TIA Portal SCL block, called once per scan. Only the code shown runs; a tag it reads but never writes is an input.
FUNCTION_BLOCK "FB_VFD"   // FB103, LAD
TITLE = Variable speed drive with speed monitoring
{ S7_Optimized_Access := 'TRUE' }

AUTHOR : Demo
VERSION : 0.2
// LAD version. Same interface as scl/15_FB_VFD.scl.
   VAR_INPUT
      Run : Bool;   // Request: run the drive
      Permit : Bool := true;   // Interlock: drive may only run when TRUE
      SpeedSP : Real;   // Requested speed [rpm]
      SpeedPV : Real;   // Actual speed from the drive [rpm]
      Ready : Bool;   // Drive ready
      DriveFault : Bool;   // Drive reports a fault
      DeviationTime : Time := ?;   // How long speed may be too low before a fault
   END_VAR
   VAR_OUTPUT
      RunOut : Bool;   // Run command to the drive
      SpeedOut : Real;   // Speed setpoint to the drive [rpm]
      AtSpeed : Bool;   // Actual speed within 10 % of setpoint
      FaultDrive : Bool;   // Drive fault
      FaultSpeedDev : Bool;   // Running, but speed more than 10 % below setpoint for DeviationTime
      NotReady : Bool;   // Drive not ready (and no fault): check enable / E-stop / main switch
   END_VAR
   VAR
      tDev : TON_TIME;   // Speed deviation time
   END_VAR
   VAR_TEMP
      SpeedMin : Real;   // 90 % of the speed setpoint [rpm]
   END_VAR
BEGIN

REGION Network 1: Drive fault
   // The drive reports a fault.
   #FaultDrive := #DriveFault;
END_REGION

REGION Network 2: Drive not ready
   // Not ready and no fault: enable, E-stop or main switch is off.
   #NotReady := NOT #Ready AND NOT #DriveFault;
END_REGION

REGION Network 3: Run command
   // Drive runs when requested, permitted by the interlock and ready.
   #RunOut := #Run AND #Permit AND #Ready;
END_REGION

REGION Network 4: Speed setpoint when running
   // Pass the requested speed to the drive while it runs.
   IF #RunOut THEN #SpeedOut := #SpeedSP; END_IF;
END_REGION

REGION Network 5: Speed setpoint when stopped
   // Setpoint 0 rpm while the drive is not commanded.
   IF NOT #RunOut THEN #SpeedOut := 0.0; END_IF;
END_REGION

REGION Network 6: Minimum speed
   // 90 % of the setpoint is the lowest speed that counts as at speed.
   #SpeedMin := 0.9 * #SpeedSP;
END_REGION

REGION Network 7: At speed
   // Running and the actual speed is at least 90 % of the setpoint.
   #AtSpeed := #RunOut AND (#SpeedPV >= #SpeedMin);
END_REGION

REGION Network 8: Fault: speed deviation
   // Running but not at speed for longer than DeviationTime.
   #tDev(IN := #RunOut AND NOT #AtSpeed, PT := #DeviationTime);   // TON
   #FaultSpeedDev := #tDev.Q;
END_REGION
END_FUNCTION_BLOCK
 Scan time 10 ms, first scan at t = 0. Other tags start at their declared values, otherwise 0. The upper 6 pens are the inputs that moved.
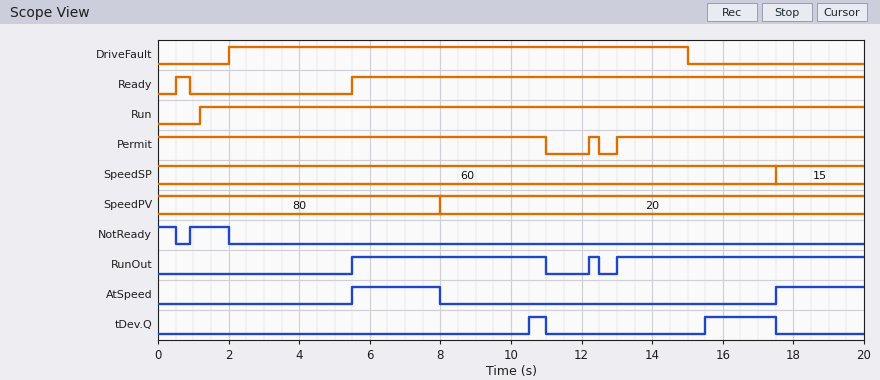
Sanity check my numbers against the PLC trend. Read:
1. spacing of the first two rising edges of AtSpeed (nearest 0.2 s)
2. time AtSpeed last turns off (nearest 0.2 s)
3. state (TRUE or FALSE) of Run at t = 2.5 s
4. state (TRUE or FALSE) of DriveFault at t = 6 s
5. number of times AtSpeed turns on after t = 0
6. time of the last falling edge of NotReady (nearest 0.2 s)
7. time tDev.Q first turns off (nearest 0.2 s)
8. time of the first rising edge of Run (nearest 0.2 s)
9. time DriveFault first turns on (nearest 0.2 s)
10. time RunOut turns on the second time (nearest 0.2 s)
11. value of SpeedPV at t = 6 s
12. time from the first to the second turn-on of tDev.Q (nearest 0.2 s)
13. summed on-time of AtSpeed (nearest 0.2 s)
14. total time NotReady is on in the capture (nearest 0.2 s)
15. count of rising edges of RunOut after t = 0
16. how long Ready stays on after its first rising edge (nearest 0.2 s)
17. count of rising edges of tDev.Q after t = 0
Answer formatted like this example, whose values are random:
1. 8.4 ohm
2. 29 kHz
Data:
1. 12.0 s
2. 8.0 s
3. TRUE
4. TRUE
5. 2
6. 2.0 s
7. 11.0 s
8. 1.2 s
9. 2.0 s
10. 12.2 s
11. 80
12. 5.0 s
13. 5.0 s
14. 1.6 s
15. 3
16. 0.4 s
17. 2
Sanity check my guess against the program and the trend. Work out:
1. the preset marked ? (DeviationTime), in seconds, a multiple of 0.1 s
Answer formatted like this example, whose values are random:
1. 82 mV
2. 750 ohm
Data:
1. 2.5 s
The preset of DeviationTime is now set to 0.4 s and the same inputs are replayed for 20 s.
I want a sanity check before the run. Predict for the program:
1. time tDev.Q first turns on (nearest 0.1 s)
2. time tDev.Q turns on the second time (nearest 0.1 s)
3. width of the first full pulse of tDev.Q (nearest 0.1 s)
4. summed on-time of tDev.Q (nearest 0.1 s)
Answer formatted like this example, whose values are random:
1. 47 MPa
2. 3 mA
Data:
1. 8.4 s
2. 13.4 s
3. 2.6 s
4. 6.7 s
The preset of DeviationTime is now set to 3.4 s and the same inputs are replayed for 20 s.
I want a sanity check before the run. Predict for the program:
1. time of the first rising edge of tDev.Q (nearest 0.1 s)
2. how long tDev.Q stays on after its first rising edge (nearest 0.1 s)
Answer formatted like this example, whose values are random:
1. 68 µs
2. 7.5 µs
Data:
1. 16.4 s
2. 1.1 s
